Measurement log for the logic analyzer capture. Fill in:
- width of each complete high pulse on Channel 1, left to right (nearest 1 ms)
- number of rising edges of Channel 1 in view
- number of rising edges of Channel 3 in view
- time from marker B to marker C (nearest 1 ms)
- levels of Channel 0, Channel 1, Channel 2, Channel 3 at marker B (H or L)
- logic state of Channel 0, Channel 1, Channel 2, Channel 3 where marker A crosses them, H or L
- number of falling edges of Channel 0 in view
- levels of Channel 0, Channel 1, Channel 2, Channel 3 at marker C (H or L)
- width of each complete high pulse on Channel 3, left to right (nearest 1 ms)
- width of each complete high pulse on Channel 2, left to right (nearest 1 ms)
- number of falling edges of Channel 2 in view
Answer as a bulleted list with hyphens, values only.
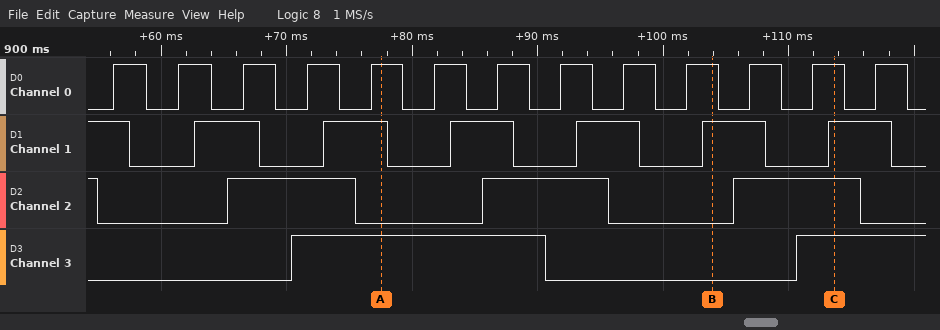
- 5 ms, 5 ms, 5 ms, 5 ms, 5 ms, 5 ms
- 6
- 2
- 10 ms
- Channel 0=H, Channel 1=H, Channel 2=L, Channel 3=L
- Channel 0=H, Channel 1=H, Channel 2=L, Channel 3=H
- 13
- Channel 0=H, Channel 1=H, Channel 2=H, Channel 3=H
- 20 ms
- 10 ms, 10 ms, 10 ms
- 4
